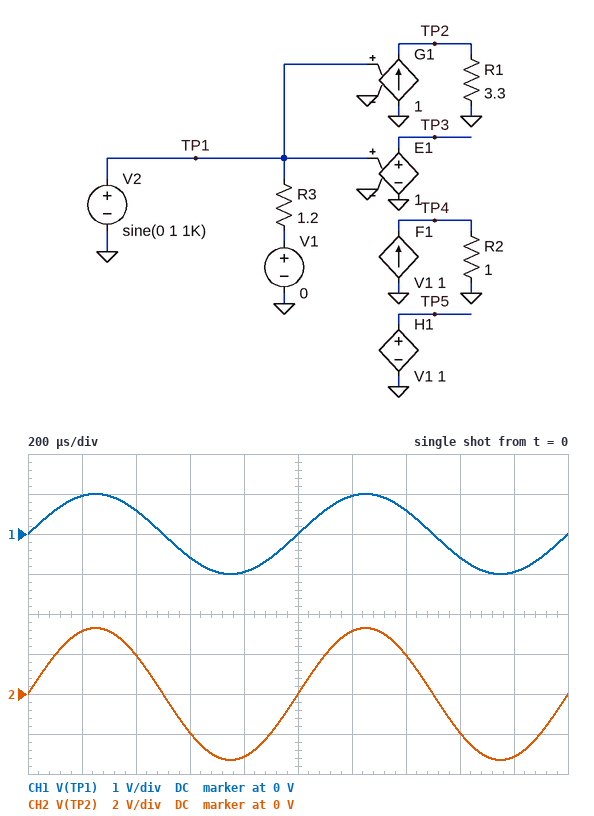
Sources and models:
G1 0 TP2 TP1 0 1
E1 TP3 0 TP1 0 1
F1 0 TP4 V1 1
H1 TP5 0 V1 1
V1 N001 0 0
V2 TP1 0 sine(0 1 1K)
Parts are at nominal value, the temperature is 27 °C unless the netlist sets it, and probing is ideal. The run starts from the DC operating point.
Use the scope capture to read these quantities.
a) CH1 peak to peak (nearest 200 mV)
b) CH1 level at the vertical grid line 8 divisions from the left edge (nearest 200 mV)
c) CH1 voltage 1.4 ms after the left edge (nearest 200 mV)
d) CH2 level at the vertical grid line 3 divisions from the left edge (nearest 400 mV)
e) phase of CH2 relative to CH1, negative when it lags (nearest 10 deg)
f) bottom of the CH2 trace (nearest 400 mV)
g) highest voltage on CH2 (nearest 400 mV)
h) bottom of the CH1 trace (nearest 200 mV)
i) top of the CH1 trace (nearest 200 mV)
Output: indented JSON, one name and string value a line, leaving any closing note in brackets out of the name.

{
  "CH1 peak to peak": "2.0 V",
  "CH1 level at the vertical grid line 8 divisions from the left edge": "-600 mV",
  "CH1 voltage 1.4 ms after the left edge": "600 mV",
  "CH2 level at the vertical grid line 3 divisions from the left edge": "-2.0 V",
  "phase of CH2 relative to CH1, negative when it lags": "0 deg",
  "bottom of the CH2 trace": "-3.2 V",
  "highest voltage on CH2": "3.2 V",
  "bottom of the CH1 trace": "-1.0 V",
  "top of the CH1 trace": "1.0 V"
}
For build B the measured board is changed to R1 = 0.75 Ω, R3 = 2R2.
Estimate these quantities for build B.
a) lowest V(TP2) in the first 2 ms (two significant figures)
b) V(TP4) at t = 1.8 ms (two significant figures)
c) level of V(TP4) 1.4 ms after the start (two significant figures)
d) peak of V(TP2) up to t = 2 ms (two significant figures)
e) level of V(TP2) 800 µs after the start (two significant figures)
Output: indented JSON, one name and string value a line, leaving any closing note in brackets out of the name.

{
  "lowest V(TP2) in the first 2 ms": "-750 mV",
  "V(TP4) at t = 1.8 ms": "-430 mV",
  "level of V(TP4) 1.4 ms after the start": "270 mV",
  "peak of V(TP2) up to t = 2 ms": "750 mV",
  "level of V(TP2) 800 µs after the start": "-710 mV"
}
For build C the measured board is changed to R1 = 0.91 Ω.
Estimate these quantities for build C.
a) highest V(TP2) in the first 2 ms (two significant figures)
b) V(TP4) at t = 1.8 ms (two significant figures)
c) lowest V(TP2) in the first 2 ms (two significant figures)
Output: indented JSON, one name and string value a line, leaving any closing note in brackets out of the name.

{
  "highest V(TP2) in the first 2 ms": "910 mV",
  "V(TP4) at t = 1.8 ms": "-790 mV",
  "lowest V(TP2) in the first 2 ms": "-910 mV"
}
